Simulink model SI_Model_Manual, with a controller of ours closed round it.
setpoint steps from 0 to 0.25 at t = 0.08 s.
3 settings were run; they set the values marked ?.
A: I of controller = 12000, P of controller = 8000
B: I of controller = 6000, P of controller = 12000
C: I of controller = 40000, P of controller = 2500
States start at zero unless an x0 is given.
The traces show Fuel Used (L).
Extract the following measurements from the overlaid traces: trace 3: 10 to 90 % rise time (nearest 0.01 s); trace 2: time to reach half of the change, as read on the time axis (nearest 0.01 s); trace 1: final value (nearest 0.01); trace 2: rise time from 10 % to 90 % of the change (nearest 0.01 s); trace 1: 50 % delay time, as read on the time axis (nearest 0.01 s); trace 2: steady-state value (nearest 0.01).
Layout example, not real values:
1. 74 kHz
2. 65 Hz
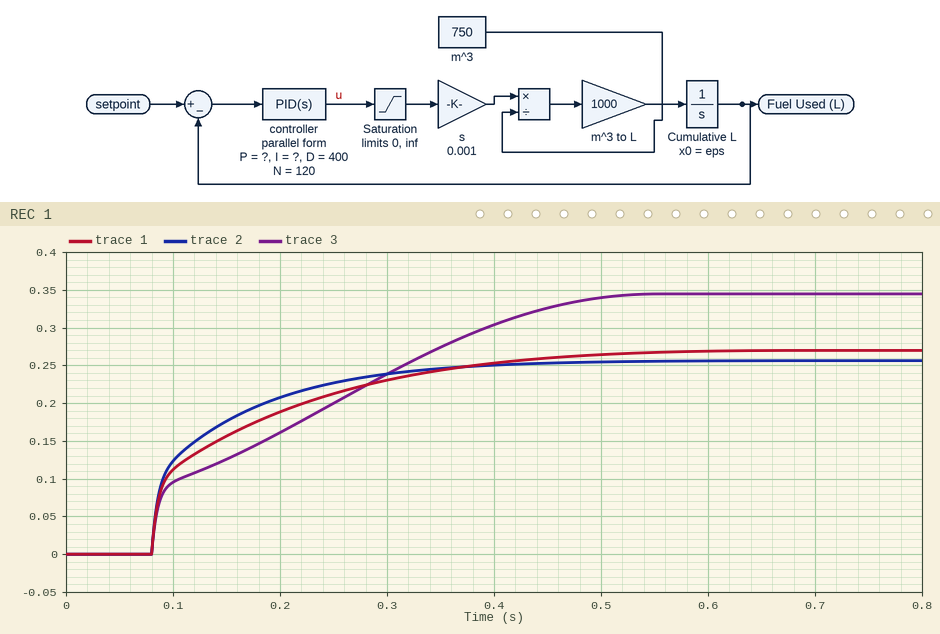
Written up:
1. 0.33 s
2. 0.10 s
3. 0.27
4. 0.18 s
5. 0.12 s
6. 0.26
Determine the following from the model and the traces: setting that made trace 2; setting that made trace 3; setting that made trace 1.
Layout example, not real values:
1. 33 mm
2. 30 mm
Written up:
1. B
2. C
3. A
